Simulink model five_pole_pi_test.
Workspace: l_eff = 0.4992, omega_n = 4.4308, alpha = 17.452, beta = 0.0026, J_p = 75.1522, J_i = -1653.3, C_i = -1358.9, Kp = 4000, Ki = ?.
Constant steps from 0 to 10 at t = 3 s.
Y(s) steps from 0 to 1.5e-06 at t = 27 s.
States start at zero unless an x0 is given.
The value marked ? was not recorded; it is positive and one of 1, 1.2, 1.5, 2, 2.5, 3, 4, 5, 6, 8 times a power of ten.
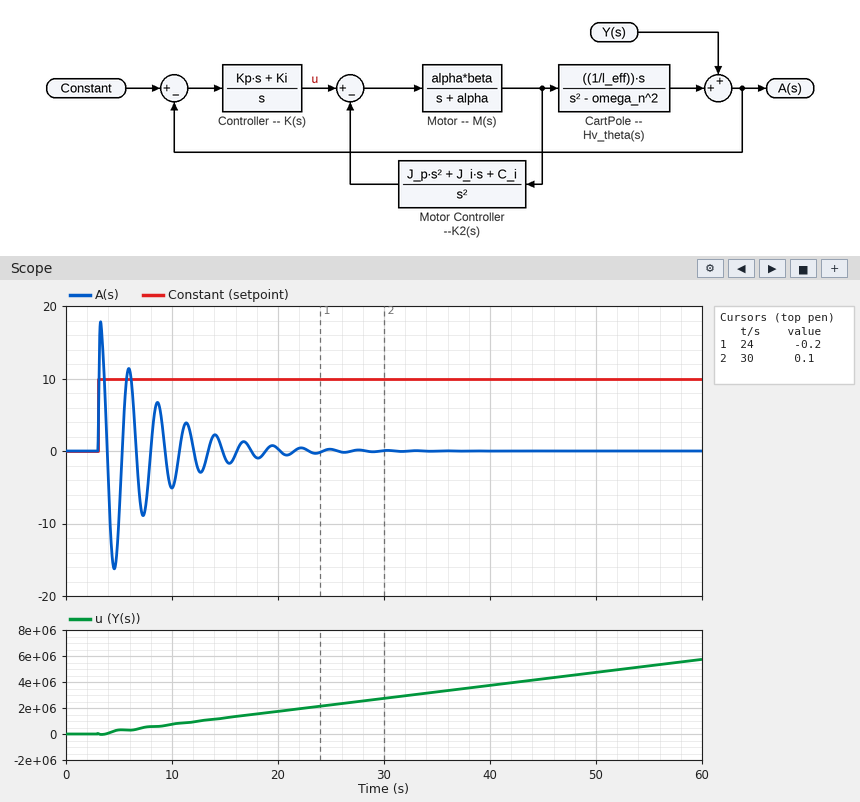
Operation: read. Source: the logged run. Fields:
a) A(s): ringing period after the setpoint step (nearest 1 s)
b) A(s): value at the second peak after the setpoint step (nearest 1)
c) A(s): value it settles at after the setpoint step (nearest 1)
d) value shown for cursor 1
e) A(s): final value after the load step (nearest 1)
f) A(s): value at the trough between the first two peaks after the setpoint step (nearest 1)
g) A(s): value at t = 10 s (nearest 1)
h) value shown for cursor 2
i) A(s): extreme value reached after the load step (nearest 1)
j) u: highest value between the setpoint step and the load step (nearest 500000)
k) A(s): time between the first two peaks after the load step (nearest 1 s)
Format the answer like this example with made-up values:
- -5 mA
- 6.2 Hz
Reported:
- 3 s
- 11
- 0
- -0.2
- 0
- -16
- -5
- 0.1
- 0
- 2500000
- 3 s
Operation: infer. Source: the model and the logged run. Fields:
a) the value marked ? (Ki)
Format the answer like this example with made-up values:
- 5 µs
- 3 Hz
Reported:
- 10000
